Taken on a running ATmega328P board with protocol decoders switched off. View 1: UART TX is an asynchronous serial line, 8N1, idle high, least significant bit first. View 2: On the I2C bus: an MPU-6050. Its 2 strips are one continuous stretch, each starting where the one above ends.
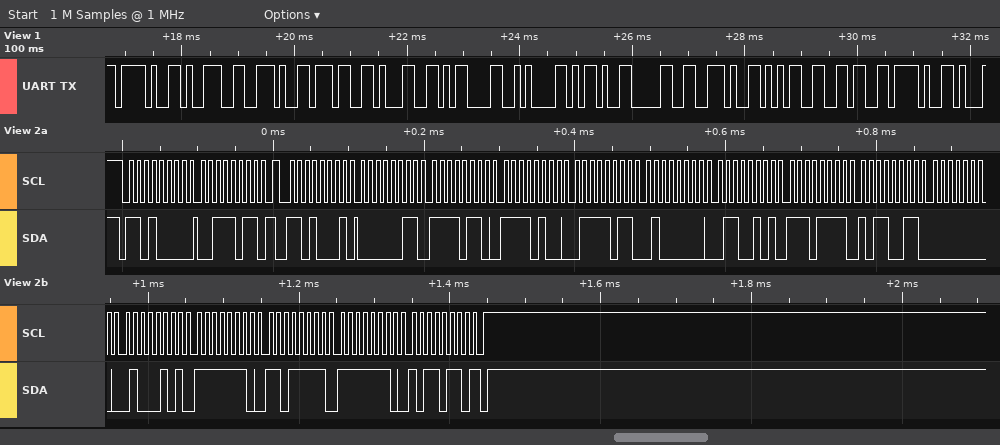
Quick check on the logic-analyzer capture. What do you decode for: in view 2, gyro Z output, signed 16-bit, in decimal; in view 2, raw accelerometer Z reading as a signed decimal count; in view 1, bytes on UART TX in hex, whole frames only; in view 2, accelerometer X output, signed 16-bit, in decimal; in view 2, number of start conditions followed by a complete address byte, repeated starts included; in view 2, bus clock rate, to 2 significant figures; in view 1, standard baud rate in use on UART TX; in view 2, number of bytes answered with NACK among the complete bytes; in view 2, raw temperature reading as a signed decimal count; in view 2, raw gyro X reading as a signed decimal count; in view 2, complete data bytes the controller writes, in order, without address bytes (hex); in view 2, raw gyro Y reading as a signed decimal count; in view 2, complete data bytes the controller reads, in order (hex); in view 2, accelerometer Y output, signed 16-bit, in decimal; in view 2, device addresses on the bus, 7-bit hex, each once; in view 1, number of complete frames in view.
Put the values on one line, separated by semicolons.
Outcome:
-330; 16485; 2F 39 2E 37 31 0D 0A 2D 30 2E 35 36 2F; 1014; 2; 100 kHz; 9600 baud; 1; -4173; 69; 3B; -289; 03 F6 F4 7B 40 65 EF B3 00 45 FE DF FE B6; -2949; 0x68; 13
